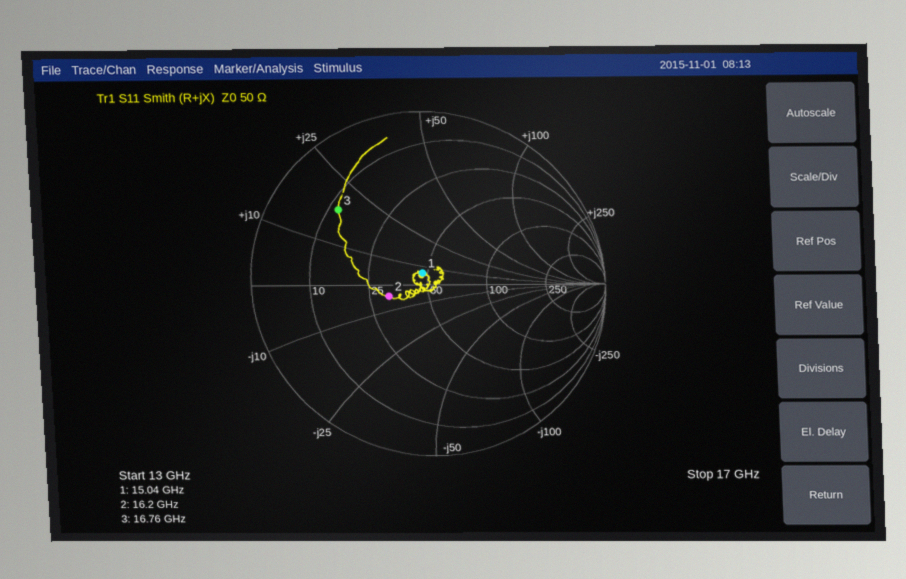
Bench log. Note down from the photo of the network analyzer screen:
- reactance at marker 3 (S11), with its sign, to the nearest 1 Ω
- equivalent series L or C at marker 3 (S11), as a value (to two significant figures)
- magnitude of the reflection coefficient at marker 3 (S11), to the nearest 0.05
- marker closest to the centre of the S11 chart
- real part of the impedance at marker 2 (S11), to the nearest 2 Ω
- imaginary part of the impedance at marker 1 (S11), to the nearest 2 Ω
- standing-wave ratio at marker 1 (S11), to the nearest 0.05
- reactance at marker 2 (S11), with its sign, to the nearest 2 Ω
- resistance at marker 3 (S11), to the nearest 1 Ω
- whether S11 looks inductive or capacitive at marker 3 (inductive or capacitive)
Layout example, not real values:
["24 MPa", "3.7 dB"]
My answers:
["+18 Ω", "170 pH", "0.65", "marker 1", "32 Ω", "+6 Ω", "1.15", "-4 Ω", "12 Ω", "inductive"]
